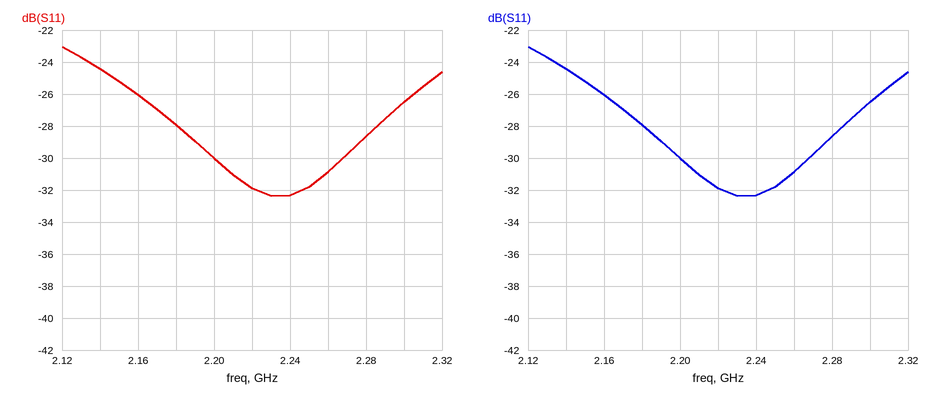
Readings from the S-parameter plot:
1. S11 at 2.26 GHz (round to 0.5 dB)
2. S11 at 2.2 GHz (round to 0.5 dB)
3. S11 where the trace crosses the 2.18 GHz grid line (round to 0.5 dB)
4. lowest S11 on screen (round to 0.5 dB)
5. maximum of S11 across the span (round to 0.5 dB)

-31.0 dB
-30.0 dB
-28.0 dB
-32.5 dB
-23.0 dB
